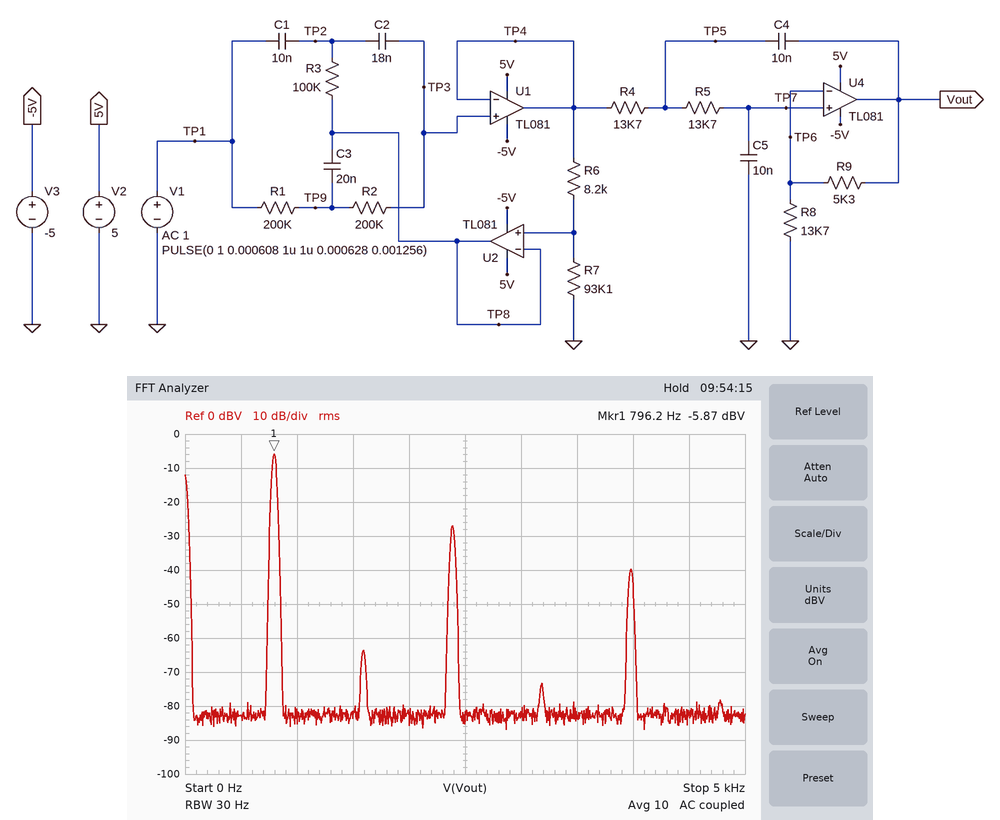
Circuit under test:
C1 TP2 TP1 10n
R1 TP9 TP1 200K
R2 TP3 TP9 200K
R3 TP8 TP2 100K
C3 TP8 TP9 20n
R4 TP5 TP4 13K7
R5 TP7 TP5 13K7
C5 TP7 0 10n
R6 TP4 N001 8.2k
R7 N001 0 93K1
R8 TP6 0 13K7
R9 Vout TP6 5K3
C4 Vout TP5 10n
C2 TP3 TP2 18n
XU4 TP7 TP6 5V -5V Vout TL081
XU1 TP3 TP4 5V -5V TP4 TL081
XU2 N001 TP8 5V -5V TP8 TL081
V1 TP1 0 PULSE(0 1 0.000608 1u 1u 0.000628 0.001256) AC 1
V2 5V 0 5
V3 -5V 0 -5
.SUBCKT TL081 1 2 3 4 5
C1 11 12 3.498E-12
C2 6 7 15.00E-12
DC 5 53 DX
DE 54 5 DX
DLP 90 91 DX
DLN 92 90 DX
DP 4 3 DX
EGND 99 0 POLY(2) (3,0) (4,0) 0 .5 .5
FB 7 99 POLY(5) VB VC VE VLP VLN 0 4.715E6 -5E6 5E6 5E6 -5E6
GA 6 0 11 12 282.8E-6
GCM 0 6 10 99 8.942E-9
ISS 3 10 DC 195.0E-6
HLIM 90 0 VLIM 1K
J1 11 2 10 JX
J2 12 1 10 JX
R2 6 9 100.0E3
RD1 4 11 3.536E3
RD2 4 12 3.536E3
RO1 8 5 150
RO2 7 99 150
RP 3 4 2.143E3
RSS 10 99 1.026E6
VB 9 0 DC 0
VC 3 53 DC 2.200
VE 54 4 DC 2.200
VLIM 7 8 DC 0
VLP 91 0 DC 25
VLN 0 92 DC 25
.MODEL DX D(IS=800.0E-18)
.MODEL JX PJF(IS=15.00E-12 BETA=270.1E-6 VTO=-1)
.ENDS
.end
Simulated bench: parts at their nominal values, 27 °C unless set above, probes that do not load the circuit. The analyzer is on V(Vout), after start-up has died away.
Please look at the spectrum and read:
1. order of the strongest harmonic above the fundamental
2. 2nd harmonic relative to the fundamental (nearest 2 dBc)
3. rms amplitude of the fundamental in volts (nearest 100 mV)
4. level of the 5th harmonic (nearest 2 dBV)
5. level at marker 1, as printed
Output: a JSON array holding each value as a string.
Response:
["3", "-58 dBc", "500 mV", "-40 dBV", "-5.87 dBV"]
